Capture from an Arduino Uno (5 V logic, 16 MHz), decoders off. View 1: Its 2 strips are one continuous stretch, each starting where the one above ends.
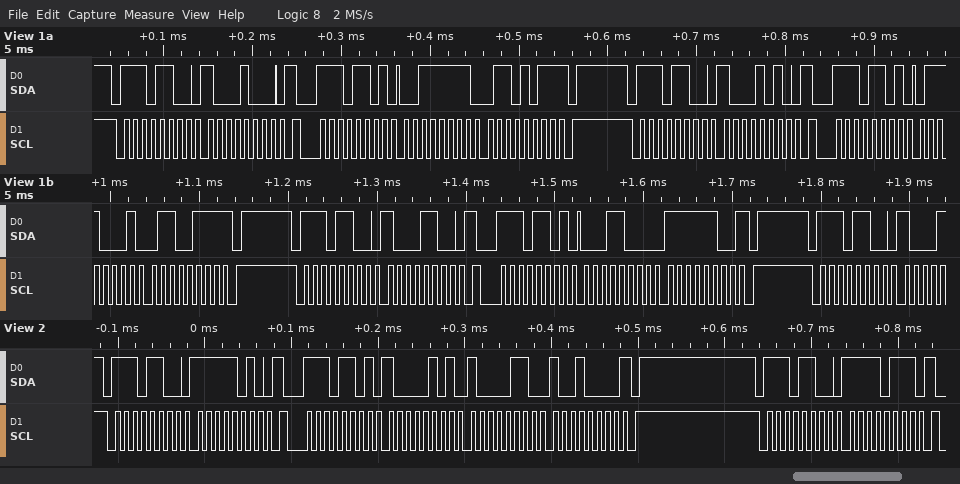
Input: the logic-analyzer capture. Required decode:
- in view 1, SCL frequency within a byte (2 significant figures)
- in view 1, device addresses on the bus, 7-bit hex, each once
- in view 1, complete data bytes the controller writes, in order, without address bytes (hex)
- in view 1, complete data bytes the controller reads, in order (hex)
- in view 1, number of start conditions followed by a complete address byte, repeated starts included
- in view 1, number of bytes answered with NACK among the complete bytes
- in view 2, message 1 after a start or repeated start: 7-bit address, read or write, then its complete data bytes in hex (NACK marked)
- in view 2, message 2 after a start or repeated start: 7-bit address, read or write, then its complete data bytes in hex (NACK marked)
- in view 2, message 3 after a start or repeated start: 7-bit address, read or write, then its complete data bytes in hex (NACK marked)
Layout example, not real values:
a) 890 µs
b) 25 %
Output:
a) 100 kHz
b) 0x76
c) 88 8A 8C
d) 3F 6B 71 67 18 FC
e) 7
f) 3
g) 0x76 write: FA
h) 0x76 read: 85 86 90 NACK
i) 0x76 write: F7
